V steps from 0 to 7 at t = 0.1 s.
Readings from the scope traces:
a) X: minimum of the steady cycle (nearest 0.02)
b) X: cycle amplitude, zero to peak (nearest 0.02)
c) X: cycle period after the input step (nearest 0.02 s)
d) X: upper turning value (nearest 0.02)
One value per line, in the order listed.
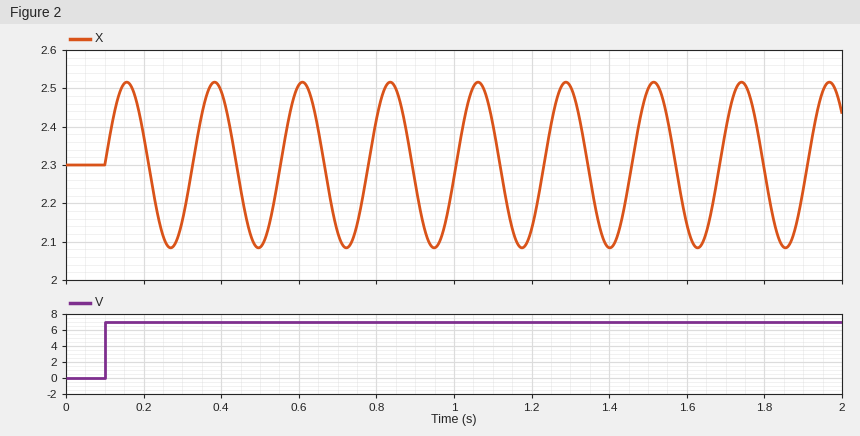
2.08
0.22
0.22 s
2.52
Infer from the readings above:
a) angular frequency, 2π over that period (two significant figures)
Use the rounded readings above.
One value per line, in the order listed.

29 rad/s
